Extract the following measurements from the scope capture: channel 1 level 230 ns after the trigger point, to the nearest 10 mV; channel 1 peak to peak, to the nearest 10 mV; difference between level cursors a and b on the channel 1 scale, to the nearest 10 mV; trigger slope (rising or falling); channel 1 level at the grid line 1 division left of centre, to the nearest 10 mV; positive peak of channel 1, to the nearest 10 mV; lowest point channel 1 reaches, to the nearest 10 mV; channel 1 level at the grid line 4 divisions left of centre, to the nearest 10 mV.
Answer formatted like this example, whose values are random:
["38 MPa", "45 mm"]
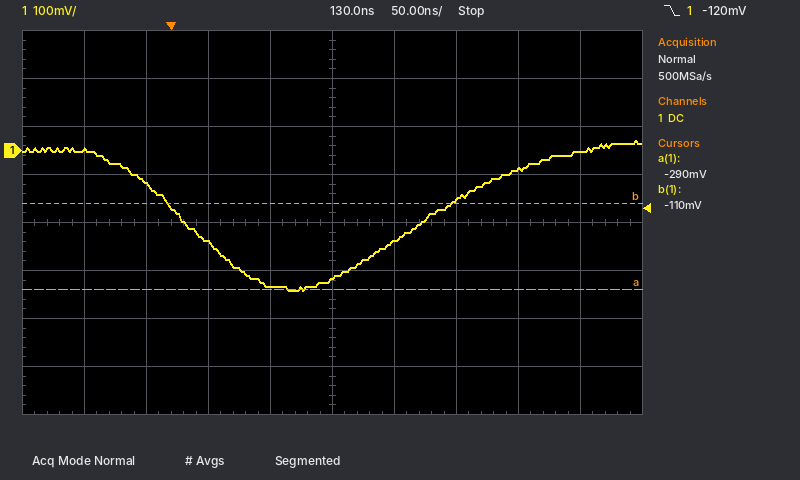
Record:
["-100 mV", "310 mV", "180 mV", "falling", "-280 mV", "20 mV", "-290 mV", "0 mV"]
